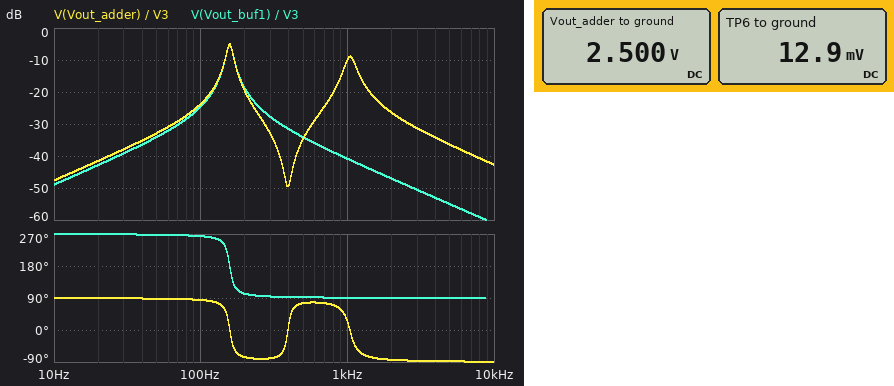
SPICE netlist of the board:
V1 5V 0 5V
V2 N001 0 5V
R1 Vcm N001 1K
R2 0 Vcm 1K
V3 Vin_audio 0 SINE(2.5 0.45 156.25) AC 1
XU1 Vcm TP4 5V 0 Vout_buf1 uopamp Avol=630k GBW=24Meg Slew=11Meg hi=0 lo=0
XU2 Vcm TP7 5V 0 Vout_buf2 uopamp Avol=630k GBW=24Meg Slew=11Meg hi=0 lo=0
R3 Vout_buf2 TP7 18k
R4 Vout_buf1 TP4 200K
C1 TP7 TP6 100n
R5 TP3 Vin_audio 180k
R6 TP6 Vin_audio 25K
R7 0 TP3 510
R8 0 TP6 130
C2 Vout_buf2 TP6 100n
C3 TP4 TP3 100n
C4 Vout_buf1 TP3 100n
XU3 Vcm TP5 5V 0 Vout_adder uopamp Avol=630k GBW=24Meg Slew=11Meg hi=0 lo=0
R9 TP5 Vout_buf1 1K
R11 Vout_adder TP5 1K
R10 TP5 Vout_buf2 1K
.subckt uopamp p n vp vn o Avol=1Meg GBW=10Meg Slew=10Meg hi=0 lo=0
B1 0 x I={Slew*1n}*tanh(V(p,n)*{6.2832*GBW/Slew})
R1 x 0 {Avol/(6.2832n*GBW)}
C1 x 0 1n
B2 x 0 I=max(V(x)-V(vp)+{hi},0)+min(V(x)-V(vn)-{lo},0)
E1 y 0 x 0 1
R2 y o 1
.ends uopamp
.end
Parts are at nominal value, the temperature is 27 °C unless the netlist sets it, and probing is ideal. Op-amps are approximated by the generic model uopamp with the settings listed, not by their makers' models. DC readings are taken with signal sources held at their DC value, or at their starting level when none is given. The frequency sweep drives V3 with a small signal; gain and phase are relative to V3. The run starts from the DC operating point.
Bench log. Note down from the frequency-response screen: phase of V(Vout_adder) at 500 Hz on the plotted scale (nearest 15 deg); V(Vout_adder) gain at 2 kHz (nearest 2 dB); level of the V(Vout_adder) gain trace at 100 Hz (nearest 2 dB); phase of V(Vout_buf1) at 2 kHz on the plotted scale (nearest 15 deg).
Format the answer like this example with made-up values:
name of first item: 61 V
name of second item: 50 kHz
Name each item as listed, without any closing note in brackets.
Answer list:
phase of V(Vout_adder) at 500 Hz on the plotted scale: 75 deg
V(Vout_adder) gain at 2 kHz: -26 dB
level of the V(Vout_adder) gain trace at 100 Hz: -24 dB
phase of V(Vout_buf1) at 2 kHz on the plotted scale: 90 deg
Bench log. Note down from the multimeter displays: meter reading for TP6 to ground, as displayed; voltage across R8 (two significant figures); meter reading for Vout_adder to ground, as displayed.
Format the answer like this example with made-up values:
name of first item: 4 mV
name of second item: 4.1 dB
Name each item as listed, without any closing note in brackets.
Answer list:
meter reading for TP6 to ground, as displayed: 12.9 mV
voltage across R8: 13 mV
meter reading for Vout_adder to ground, as displayed: 2.500 V
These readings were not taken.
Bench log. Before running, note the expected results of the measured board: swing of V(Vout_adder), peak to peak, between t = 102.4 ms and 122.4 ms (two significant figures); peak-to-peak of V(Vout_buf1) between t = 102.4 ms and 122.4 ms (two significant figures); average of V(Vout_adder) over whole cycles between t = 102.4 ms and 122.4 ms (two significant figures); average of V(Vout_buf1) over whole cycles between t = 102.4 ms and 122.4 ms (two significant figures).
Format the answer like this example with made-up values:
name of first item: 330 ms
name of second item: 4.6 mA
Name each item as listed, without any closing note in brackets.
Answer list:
swing of V(Vout_adder), peak to peak, between t = 102.4 ms and 122.4 ms: 490 mV
peak-to-peak of V(Vout_buf1) between t = 102.4 ms and 122.4 ms: 490 mV
average of V(Vout_adder) over whole cycles between t = 102.4 ms and 122.4 ms: 2.5 V
average of V(Vout_buf1) over whole cycles between t = 102.4 ms and 122.4 ms: 2.5 V
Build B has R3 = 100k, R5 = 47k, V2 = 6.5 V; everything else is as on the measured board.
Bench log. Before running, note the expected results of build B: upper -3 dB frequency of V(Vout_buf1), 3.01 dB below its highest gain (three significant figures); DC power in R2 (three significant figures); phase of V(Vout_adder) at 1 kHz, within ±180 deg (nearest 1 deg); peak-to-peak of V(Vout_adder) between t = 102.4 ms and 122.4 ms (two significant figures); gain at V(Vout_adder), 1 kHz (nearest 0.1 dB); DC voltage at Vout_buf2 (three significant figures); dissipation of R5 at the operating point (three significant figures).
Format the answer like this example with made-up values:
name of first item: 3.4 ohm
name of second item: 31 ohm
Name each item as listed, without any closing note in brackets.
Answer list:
upper -3 dB frequency of V(Vout_buf1), 3.01 dB below its highest gain: 167 Hz
DC power in R2: 10.6 mW
phase of V(Vout_adder) at 1 kHz, within ±180 deg: -88 deg
peak-to-peak of V(Vout_adder) between t = 102.4 ms and 122.4 ms: 1.9 V
gain at V(Vout_adder), 1 kHz: -18.9 dB
DC voltage at Vout_buf2: 3.25 V
dissipation of R5 at the operating point: 130 µW
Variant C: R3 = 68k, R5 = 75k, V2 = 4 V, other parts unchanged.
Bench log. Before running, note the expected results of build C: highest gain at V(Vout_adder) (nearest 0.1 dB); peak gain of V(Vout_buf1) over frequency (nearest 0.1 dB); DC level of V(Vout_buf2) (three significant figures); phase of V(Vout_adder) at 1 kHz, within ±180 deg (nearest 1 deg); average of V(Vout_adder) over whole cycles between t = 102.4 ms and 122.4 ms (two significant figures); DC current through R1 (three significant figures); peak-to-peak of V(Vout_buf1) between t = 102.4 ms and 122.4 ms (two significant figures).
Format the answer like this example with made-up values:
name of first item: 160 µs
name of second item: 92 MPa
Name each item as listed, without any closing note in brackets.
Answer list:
highest gain at V(Vout_adder): 2.7 dB
peak gain of V(Vout_buf1) over frequency: 2.5 dB
DC level of V(Vout_buf2): 2.00 V
phase of V(Vout_adder) at 1 kHz, within ±180 deg: -87 deg
average of V(Vout_adder) over whole cycles between t = 102.4 ms and 122.4 ms: 2.0 V
DC current through R1: 2.00 mA
peak-to-peak of V(Vout_buf1) between t = 102.4 ms and 122.4 ms: 1.2 V
